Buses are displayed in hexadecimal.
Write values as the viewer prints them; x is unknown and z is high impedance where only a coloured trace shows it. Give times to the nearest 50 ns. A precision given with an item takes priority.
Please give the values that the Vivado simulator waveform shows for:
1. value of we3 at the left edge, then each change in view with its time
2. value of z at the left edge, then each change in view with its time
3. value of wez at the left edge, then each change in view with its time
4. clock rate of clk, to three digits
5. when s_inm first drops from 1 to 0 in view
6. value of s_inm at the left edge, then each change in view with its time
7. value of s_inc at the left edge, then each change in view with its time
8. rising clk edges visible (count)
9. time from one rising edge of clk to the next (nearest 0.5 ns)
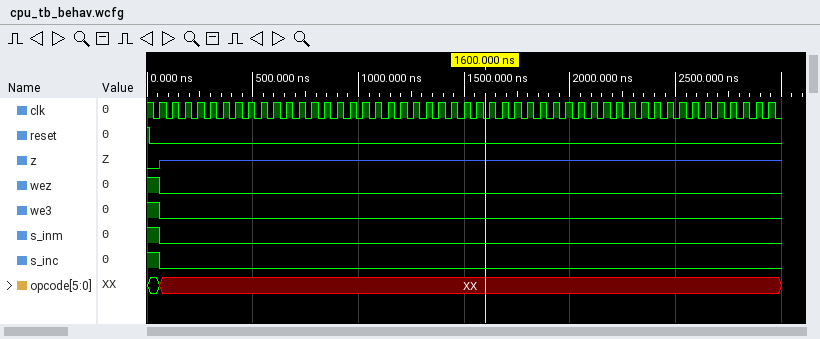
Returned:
1, 0 at 50 ns
0, z at 50 ns
1, 0 at 50 ns
16.7 MHz
50 ns
1, 0 at 50 ns
1, 0 at 50 ns
49
60 ns
